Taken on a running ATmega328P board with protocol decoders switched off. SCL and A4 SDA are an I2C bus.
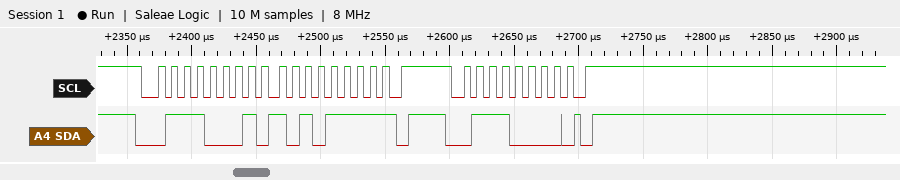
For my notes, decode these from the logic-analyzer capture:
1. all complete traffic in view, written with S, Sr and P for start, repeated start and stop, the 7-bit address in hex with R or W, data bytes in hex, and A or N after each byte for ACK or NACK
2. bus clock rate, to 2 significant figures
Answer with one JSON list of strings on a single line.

["S 38R A AF N P S 38W A P", "100 kHz"]
